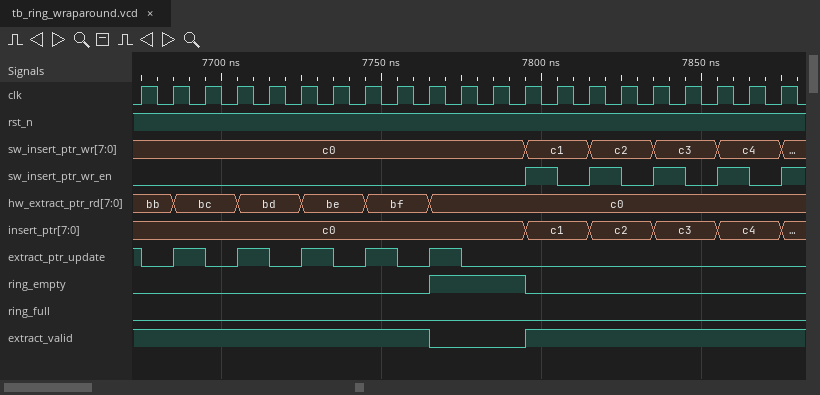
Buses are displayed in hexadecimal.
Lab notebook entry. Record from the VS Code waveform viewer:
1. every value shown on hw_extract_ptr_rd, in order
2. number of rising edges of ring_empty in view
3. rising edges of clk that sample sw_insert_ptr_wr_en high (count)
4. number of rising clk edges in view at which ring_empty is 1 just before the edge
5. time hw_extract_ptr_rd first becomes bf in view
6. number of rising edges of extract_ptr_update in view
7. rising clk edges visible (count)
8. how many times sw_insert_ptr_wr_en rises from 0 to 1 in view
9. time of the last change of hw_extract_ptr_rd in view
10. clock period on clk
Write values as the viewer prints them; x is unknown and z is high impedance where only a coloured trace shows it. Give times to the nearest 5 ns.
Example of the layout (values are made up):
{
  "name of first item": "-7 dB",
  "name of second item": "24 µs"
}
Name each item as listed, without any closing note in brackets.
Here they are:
{
  "every value shown on hw_extract_ptr_rd, in order": "bb, bc, bd, be, bf, c0",
  "number of rising edges of ring_empty in view": "1",
  "rising edges of clk that sample sw_insert_ptr_wr_en high": "4",
  "number of rising clk edges in view at which ring_empty is 1 just before the edge": "3",
  "time hw_extract_ptr_rd first becomes bf in view": "7745 ns",
  "number of rising edges of extract_ptr_update in view": "5",
  "rising clk edges visible": "21",
  "how many times sw_insert_ptr_wr_en rises from 0 to 1 in view": "5",
  "time of the last change of hw_extract_ptr_rd in view": "7765 ns",
  "clock period on clk": "10 ns"
}
